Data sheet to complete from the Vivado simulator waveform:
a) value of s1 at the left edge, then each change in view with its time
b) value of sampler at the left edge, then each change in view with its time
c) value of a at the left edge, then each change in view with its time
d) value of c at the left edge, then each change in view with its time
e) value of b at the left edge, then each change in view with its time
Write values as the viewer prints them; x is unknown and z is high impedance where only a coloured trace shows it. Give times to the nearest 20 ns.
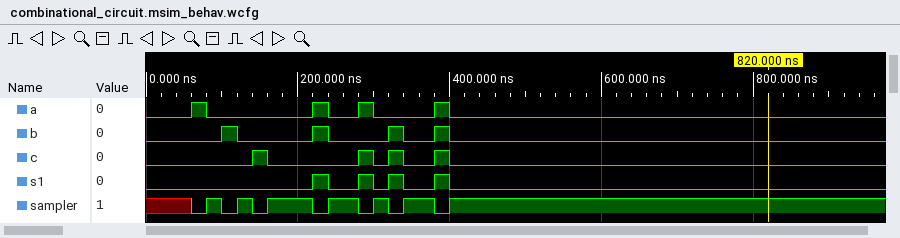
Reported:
0, 1 at 220 ns, 0 at 240 ns, 1 at 280 ns, 0 at 300 ns, 1 at 320 ns, 0 at 340 ns, 1 at 380 ns, 0 at 400 ns
x, 0 at 60 ns, 1 at 80 ns, 0 at 100 ns, 1 at 120 ns, 0 at 140 ns, 1 at 160 ns, 0 at 220 ns, 1 at 240 ns, 0 at 280 ns, 1 at 300 ns, 0 at 320 ns, 1 at 340 ns, 0 at 380 ns, 1 at 400 ns
0, 1 at 60 ns, 0 at 80 ns, 1 at 220 ns, 0 at 240 ns, 1 at 280 ns, 0 at 300 ns, 1 at 380 ns, 0 at 400 ns
0, 1 at 140 ns, 0 at 160 ns, 1 at 280 ns, 0 at 300 ns, 1 at 320 ns, 0 at 340 ns, 1 at 380 ns, 0 at 400 ns
0, 1 at 100 ns, 0 at 120 ns, 1 at 220 ns, 0 at 240 ns, 1 at 320 ns, 0 at 340 ns, 1 at 380 ns, 0 at 400 ns
